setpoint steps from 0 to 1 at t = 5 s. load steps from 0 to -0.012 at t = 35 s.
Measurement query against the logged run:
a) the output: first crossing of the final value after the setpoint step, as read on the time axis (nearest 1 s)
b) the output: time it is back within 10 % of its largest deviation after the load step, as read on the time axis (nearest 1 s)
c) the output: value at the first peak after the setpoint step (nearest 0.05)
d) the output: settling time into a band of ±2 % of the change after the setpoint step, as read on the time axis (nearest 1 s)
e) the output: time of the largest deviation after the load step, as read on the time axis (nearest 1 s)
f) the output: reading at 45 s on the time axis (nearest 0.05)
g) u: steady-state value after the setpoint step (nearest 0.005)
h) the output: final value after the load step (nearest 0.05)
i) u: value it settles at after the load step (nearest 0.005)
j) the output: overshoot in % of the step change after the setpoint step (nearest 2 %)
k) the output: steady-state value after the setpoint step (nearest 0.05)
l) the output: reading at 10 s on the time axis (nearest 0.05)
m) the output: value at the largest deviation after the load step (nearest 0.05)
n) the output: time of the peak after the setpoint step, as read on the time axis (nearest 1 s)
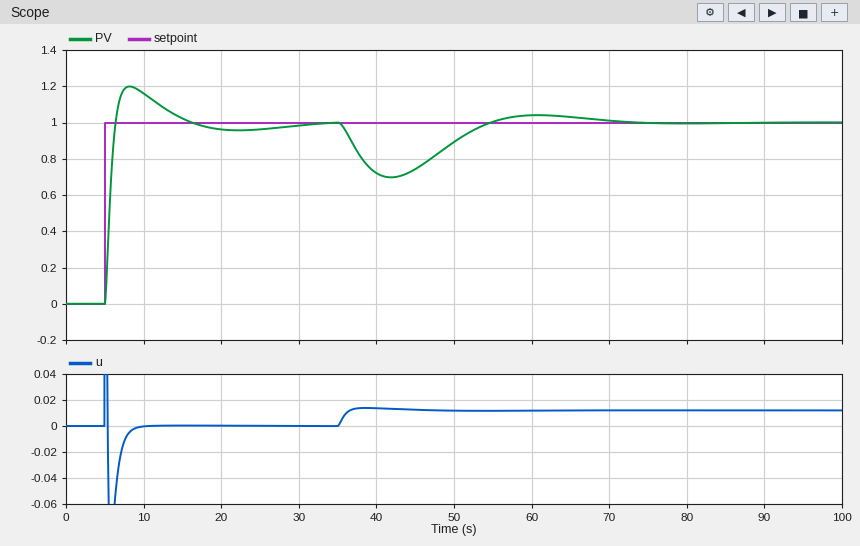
6 s
65 s
1.20
29 s
42 s
0.75
0.000
1.00
0.010
20 %
1.00
1.15
0.70
8 s
